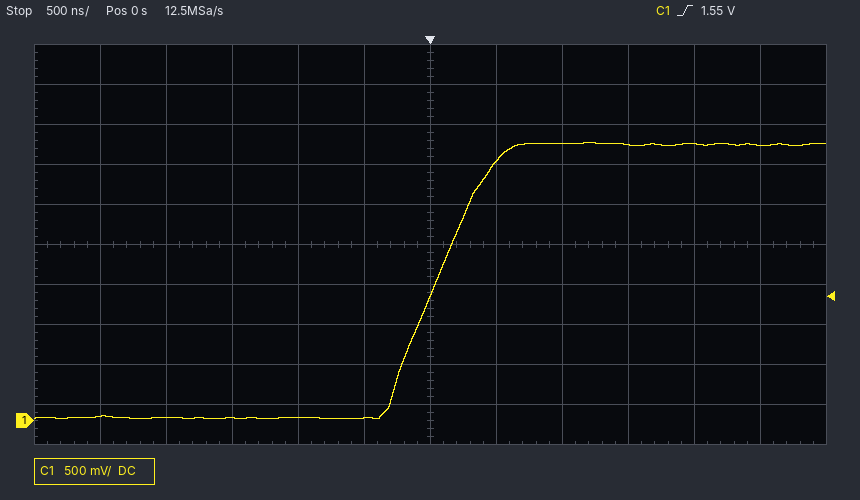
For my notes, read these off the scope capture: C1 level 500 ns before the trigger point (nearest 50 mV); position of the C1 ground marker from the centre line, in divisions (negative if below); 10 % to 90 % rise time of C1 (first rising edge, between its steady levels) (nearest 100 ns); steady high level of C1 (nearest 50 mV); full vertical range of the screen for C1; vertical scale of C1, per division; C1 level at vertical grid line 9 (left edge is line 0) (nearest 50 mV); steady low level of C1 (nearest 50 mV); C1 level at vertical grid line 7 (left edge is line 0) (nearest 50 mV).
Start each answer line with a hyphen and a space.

- 50 mV
- -4.4 div
- 700 ns
- 3.45 V
- 5 V
- 500 mV
- 3.45 V
- 50 mV
- 3.25 V
